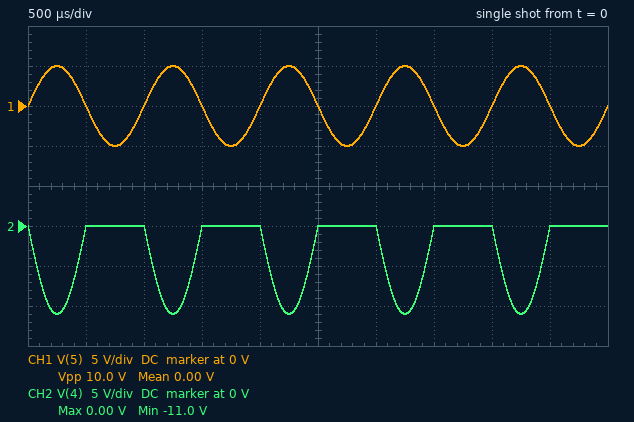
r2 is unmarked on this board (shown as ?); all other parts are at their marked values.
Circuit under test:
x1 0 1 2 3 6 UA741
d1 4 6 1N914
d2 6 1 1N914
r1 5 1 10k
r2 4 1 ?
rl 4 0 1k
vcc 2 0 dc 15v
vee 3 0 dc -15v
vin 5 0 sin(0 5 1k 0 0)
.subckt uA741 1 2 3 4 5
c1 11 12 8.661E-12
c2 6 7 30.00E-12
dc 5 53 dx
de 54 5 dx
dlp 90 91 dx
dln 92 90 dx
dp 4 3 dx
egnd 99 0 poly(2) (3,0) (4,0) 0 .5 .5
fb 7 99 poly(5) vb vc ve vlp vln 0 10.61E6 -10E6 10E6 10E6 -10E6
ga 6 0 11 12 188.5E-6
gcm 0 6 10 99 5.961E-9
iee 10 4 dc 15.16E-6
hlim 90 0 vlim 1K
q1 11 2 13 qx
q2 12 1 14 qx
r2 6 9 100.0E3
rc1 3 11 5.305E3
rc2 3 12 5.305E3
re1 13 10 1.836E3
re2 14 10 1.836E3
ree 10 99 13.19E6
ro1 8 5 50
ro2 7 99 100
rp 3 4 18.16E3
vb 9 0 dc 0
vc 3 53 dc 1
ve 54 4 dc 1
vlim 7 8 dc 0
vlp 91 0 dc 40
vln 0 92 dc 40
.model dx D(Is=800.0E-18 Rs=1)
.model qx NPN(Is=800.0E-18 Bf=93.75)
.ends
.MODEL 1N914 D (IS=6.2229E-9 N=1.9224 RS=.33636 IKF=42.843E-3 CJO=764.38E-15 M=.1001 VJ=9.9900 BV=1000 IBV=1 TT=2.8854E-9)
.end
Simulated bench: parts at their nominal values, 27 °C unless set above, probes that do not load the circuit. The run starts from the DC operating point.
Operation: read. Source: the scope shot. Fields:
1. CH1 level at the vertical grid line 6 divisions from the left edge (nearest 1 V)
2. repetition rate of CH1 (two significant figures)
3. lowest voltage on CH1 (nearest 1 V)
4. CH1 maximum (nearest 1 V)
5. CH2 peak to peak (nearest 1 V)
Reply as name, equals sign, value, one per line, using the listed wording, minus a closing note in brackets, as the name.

CH1 level at the vertical grid line 6 divisions from the left edge = 0 V
repetition rate of CH1 = 1.0 kHz
lowest voltage on CH1 = -5 V
CH1 maximum = 5 V
CH2 peak to peak = 11 V
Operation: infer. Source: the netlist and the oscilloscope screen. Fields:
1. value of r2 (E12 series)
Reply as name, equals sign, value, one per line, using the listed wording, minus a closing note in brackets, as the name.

value of r2 = 22 kΩ
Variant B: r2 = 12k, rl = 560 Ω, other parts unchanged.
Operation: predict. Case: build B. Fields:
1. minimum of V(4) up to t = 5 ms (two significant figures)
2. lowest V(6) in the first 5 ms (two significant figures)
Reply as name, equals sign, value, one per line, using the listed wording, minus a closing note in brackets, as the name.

minimum of V(4) up to t = 5 ms = -6.0 V
lowest V(6) in the first 5 ms = -6.7 V
